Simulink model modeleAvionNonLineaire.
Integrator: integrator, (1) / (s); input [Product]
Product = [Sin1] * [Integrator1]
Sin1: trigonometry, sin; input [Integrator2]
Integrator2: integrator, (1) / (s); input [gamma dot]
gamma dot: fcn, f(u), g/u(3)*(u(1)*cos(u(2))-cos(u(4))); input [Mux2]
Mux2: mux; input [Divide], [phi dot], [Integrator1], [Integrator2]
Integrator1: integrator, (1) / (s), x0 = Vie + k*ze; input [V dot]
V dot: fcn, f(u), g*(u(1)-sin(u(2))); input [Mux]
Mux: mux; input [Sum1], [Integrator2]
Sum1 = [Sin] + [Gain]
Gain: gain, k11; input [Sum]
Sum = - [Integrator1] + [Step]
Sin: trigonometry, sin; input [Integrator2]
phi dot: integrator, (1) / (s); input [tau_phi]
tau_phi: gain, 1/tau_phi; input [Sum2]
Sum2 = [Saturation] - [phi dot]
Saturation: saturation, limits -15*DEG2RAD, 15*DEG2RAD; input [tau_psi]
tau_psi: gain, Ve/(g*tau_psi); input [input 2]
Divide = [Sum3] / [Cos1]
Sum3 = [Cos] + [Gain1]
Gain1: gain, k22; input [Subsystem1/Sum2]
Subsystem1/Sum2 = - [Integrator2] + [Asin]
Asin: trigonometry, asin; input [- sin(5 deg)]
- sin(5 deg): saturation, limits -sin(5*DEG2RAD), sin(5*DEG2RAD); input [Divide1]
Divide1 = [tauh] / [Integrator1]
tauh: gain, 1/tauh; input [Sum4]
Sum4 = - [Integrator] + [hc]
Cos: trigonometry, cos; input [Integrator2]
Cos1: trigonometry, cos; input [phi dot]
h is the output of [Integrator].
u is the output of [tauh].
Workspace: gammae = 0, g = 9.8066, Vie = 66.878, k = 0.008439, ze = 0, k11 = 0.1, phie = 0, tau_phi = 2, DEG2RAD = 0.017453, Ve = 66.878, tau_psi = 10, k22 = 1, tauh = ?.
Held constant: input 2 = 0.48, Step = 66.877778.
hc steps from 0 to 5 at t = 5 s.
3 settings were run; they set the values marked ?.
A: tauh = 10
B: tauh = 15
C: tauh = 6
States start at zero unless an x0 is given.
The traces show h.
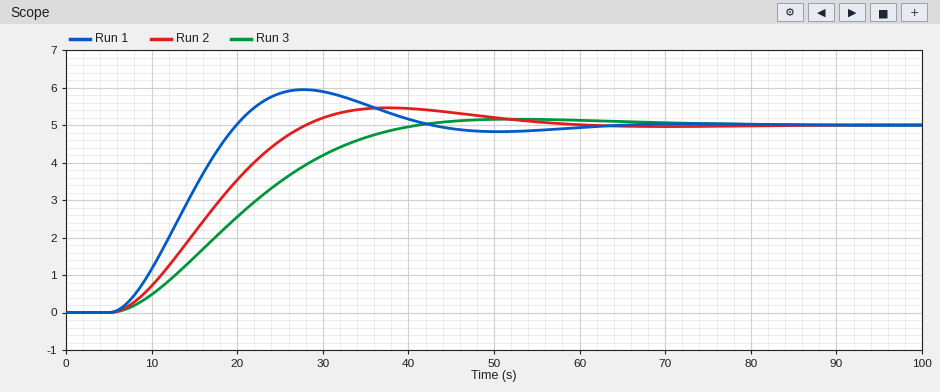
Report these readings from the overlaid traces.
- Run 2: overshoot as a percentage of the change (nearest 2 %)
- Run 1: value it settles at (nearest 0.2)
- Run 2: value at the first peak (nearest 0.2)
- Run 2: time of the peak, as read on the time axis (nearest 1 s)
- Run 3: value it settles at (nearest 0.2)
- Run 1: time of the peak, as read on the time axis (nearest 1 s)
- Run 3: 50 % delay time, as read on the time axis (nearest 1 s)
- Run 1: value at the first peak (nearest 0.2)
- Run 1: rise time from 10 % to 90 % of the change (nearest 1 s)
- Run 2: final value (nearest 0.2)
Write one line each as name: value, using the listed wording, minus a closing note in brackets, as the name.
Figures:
Run 2: overshoot as a percentage of the change: 10 %
Run 1: value it settles at: 5.0
Run 2: value at the first peak: 5.4
Run 2: time of the peak, as read on the time axis: 38 s
Run 3: value it settles at: 5.0
Run 1: time of the peak, as read on the time axis: 28 s
Run 3: 50 % delay time, as read on the time axis: 20 s
Run 1: value at the first peak: 6.0
Run 1: rise time from 10 % to 90 % of the change: 10 s
Run 2: final value: 5.0
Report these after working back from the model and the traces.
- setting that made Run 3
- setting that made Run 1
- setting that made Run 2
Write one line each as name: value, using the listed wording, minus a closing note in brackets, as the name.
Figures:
setting that made Run 3: B
setting that made Run 1: C
setting that made Run 2: A
